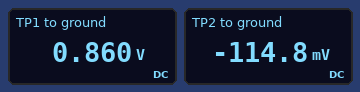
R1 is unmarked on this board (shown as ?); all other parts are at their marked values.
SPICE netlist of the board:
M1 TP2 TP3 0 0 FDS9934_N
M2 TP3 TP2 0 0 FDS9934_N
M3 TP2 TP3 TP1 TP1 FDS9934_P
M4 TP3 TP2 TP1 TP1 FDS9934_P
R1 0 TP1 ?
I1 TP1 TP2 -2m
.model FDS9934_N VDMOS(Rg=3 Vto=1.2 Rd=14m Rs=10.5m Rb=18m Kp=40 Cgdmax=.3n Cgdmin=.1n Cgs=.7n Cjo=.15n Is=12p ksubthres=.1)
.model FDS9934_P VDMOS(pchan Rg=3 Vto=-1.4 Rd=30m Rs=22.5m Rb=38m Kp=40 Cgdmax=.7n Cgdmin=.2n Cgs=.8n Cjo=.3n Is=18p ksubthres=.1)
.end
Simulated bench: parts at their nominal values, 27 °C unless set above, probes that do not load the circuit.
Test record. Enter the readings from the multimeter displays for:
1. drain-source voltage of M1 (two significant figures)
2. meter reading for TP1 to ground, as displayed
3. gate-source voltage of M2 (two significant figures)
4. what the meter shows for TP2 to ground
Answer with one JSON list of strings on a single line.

["-110 mV", "0.860 V", "-110 mV", "-114.8 mV"]
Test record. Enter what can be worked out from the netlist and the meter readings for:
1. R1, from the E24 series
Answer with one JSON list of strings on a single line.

["430 Ω"]
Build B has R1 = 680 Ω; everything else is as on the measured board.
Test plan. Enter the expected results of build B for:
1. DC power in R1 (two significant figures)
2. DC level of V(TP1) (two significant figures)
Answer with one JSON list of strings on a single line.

["2.7 mW", "1.4 V"]
